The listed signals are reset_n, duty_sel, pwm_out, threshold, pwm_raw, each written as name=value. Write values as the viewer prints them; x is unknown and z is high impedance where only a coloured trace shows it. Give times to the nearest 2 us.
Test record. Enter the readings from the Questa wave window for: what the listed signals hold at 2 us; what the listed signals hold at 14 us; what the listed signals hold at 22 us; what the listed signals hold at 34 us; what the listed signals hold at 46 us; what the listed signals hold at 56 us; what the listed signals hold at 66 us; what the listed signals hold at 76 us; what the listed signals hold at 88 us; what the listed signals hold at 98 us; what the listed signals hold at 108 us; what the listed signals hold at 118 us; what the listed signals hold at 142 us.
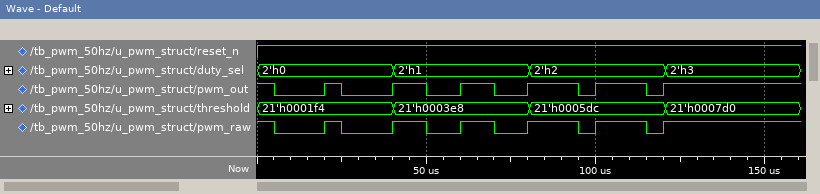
reset_n=1, duty_sel=2'h0, pwm_out=1, threshold=21'h0001f4, pwm_raw=1
reset_n=1, duty_sel=2'h0, pwm_out=0, threshold=21'h0001f4, pwm_raw=0
reset_n=1, duty_sel=2'h0, pwm_out=1, threshold=21'h0001f4, pwm_raw=1
reset_n=1, duty_sel=2'h0, pwm_out=0, threshold=21'h0001f4, pwm_raw=0
reset_n=1, duty_sel=2'h1, pwm_out=1, threshold=21'h0003e8, pwm_raw=1
reset_n=1, duty_sel=2'h1, pwm_out=0, threshold=21'h0003e8, pwm_raw=0
reset_n=1, duty_sel=2'h1, pwm_out=1, threshold=21'h0003e8, pwm_raw=1
reset_n=1, duty_sel=2'h1, pwm_out=0, threshold=21'h0003e8, pwm_raw=0
reset_n=1, duty_sel=2'h2, pwm_out=1, threshold=21'h0005dc, pwm_raw=1
reset_n=1, duty_sel=2'h2, pwm_out=0, threshold=21'h0005dc, pwm_raw=0
reset_n=1, duty_sel=2'h2, pwm_out=1, threshold=21'h0005dc, pwm_raw=1
reset_n=1, duty_sel=2'h2, pwm_out=0, threshold=21'h0005dc, pwm_raw=0
reset_n=1, duty_sel=2'h3, pwm_out=1, threshold=21'h0007d0, pwm_raw=1
